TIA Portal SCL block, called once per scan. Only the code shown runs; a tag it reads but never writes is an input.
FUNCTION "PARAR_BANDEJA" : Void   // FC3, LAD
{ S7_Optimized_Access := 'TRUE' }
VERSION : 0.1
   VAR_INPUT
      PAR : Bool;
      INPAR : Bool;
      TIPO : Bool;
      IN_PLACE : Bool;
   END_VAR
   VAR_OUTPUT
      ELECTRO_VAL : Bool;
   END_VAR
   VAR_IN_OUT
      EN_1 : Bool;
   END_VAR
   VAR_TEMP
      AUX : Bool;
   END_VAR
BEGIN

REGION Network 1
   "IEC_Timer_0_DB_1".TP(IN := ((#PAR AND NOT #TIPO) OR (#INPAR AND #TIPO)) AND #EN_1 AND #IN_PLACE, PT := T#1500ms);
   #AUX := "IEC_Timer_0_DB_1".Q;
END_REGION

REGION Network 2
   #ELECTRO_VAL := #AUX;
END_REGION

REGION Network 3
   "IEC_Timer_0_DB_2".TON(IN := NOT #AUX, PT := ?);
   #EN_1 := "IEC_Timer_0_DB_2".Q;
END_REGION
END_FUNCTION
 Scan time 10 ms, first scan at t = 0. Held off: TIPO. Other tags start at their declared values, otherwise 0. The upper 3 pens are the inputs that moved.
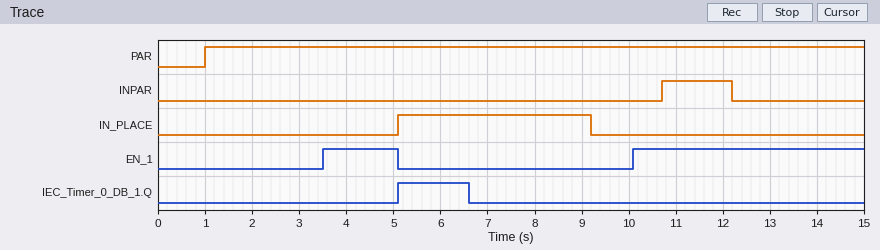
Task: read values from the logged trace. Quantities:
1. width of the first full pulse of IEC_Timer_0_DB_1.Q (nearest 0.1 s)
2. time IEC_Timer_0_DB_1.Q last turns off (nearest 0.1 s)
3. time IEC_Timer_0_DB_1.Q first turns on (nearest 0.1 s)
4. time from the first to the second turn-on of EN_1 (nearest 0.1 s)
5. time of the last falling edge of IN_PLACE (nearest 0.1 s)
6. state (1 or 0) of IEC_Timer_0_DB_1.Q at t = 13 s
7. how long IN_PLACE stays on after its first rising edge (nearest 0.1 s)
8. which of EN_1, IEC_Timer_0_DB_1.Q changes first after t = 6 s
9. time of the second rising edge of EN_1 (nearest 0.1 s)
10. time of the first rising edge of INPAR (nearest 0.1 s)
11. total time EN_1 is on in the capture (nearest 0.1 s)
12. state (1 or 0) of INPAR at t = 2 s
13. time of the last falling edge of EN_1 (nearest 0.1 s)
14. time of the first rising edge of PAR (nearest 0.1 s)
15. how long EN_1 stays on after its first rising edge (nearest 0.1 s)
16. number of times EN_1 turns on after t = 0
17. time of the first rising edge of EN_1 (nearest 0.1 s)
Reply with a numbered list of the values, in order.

1. 1.5 s
2. 6.6 s
3. 5.1 s
4. 6.6 s
5. 9.2 s
6. 0
7. 4.1 s
8. IEC_Timer_0_DB_1.Q
9. 10.1 s
10. 10.7 s
11. 6.5 s
12. 0
13. 5.1 s
14. 1.0 s
15. 1.6 s
16. 2
17. 3.5 s
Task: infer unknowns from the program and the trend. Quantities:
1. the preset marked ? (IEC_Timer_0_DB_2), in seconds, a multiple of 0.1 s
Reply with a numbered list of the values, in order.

1. 3.5 s
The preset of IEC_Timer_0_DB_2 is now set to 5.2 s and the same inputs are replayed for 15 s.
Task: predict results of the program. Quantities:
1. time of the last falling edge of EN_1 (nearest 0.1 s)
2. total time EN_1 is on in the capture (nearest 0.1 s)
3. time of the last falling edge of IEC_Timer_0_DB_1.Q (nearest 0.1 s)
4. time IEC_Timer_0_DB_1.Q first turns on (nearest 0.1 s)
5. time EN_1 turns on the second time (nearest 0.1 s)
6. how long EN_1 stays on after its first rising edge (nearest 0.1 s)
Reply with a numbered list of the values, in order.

1. 5.2 s
2. 3.1 s
3. 6.7 s
4. 5.2 s
5. 11.9 s
6. 0.0 s
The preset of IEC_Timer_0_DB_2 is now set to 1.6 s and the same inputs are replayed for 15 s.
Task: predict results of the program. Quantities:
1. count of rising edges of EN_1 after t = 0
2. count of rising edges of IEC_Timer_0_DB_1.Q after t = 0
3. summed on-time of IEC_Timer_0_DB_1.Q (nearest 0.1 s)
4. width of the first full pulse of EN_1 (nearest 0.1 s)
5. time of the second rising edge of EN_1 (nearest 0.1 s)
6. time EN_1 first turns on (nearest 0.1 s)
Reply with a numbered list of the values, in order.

1. 3
2. 2
3. 3.0 s
4. 3.5 s
5. 8.2 s
6. 1.6 s
